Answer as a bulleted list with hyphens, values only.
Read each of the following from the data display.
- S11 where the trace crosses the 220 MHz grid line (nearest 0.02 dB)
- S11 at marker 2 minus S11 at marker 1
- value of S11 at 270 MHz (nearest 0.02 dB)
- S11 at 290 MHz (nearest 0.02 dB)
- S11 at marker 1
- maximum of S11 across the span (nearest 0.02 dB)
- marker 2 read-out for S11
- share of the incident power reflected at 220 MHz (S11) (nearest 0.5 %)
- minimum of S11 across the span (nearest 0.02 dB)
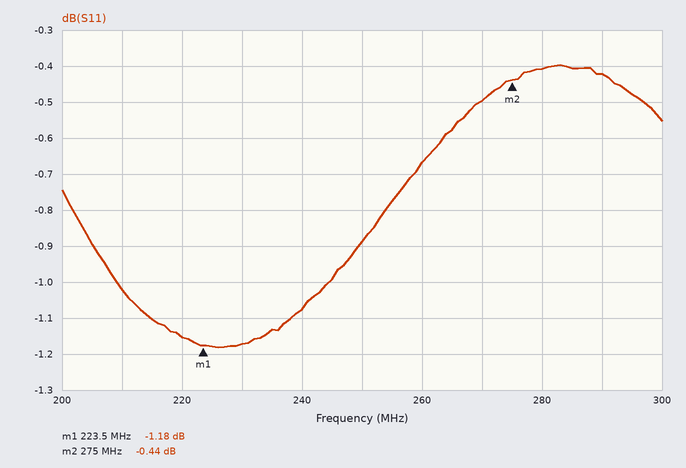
- -1.16 dB
- 0.74 dB
- -0.50 dB
- -0.42 dB
- -1.18 dB
- -0.40 dB
- -0.44 dB
- 76.5 %
- -1.18 dB
